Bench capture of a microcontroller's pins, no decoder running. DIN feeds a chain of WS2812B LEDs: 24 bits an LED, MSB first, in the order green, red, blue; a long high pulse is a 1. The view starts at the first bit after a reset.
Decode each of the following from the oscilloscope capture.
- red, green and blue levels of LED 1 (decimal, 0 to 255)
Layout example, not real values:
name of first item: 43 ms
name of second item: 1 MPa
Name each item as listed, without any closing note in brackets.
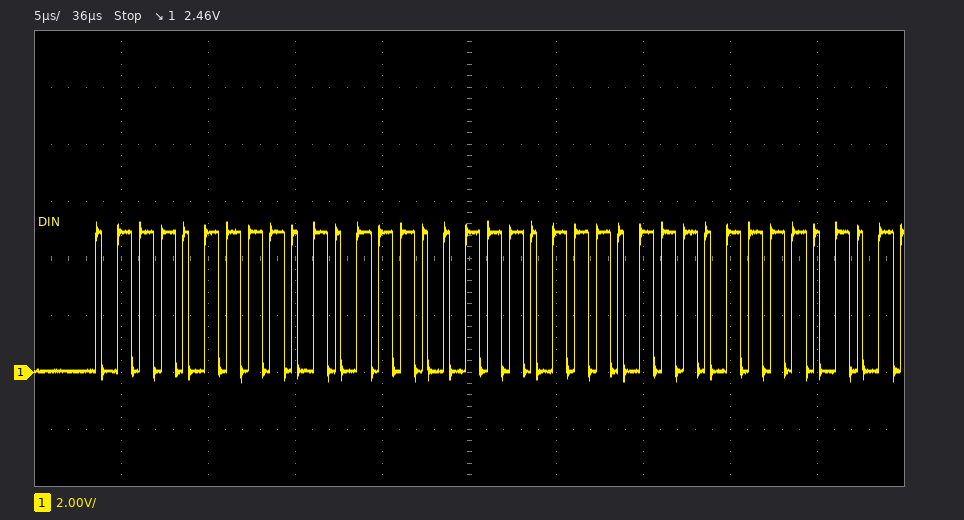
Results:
red, green and blue levels of LED 1: 174, 119, 119
